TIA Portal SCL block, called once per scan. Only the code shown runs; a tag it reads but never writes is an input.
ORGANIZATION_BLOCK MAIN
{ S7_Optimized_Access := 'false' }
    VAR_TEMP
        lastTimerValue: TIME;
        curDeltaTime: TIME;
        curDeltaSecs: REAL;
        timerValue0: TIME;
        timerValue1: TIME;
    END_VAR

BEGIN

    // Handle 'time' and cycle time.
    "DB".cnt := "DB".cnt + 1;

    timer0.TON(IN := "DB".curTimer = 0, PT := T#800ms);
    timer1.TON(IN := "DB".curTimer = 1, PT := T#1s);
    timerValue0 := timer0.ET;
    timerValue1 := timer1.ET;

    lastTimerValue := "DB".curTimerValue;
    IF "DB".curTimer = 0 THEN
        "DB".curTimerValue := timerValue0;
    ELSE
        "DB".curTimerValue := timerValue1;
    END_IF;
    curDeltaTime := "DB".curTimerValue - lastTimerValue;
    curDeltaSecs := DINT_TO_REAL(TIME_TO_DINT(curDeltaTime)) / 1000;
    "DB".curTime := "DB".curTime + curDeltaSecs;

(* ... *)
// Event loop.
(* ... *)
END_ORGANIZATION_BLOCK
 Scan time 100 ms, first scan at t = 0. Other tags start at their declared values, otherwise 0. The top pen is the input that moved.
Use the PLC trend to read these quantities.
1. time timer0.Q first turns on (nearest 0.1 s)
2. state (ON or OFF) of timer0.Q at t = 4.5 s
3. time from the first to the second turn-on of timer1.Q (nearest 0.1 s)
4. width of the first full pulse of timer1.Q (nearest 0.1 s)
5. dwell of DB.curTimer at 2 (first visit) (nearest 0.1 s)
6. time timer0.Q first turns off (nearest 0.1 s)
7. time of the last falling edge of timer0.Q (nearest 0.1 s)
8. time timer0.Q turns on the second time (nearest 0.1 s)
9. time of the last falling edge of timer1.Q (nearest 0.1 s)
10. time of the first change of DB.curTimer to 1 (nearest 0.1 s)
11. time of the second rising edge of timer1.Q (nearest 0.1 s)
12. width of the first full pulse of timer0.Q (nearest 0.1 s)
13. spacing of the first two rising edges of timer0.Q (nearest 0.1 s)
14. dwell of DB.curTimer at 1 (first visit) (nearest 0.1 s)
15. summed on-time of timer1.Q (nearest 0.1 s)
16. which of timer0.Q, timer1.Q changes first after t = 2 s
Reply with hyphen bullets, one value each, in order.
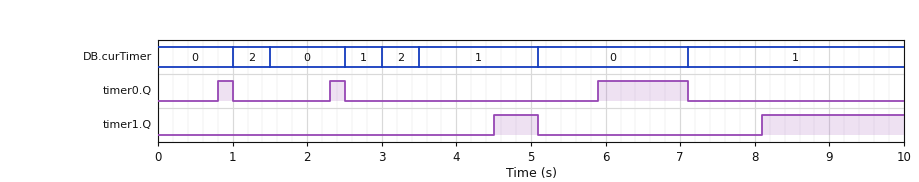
- 0.8 s
- OFF
- 3.6 s
- 0.6 s
- 0.5 s
- 1.0 s
- 7.1 s
- 2.3 s
- 5.1 s
- 2.5 s
- 8.1 s
- 0.2 s
- 1.5 s
- 0.5 s
- 2.5 s
- timer0.Q
